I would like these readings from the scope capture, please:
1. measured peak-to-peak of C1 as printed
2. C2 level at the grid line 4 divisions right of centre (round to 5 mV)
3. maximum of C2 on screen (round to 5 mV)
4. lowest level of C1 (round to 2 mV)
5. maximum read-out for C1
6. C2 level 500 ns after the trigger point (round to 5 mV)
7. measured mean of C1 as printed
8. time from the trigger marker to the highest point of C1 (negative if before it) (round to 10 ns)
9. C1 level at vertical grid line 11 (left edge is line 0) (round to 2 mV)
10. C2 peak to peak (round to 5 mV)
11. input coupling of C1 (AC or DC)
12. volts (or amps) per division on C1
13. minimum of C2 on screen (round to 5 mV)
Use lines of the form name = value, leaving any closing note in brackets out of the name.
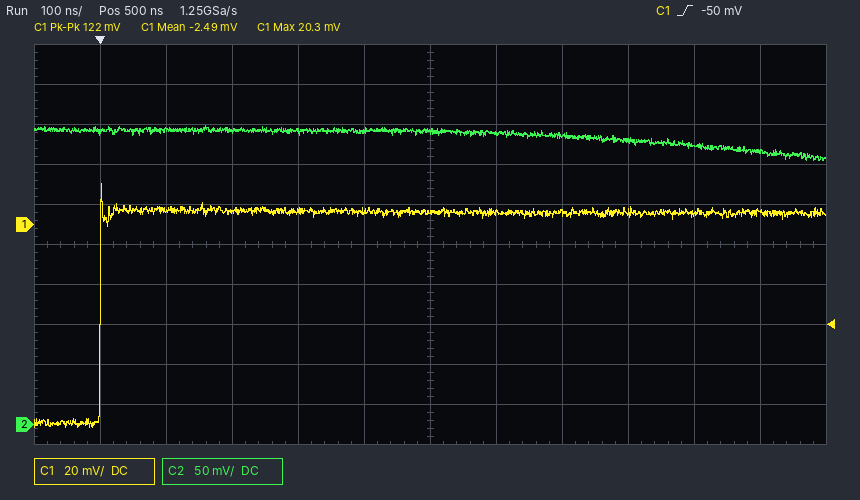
measured peak-to-peak of C1 as printed = 122 mV
C2 level at the grid line 4 divisions right of centre = 350 mV
maximum of C2 on screen = 375 mV
lowest level of C1 = -102 mV
maximum read-out for C1 = 20.3 mV
C2 level 500 ns after the trigger point = 365 mV
measured mean of C1 as printed = -2.49 mV
time from the trigger marker to the highest point of C1 (negative if before it) = 0 ns
C1 level at vertical grid line 11 (left edge is line 0) = 6 mV
C2 peak to peak = 45 mV
input coupling of C1 = DC
volts (or amps) per division on C1 = 20 mV
minimum of C2 on screen = 330 mV
